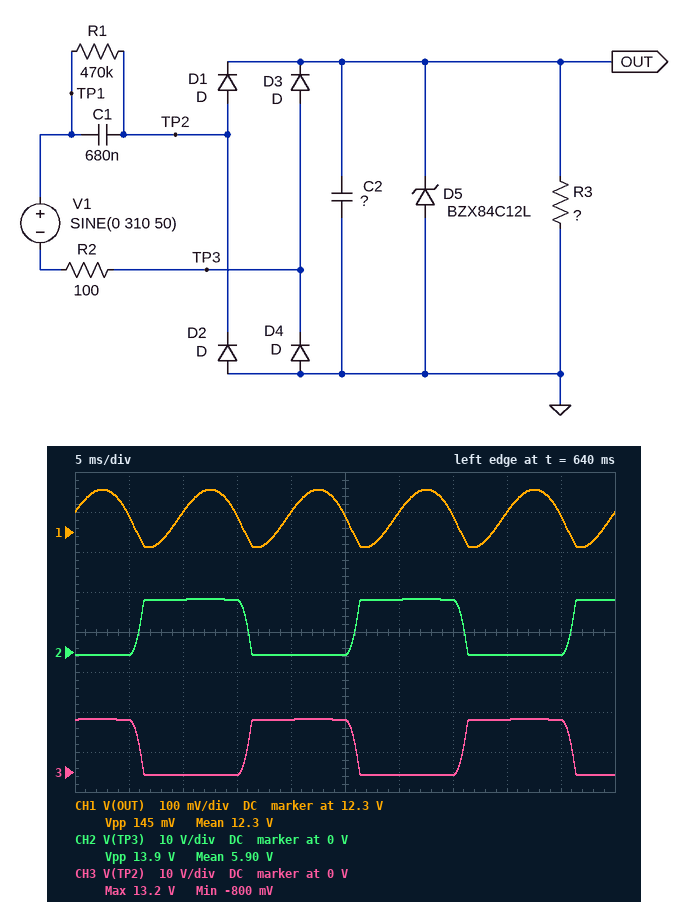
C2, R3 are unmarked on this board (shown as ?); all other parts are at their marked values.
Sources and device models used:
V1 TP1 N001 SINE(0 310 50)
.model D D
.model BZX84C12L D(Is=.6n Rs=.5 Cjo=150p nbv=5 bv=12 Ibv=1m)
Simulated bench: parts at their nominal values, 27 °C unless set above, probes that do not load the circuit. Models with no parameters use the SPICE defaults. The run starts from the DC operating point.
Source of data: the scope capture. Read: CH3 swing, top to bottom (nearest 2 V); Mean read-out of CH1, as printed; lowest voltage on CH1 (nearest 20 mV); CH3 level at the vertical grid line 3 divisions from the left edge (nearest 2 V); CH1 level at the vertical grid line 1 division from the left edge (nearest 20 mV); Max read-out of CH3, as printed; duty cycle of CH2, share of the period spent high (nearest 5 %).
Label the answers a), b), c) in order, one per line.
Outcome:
a) 14 V
b) 12.3 V
c) 12.26 V
d) 0 V
e) 12.34 V
f) 13.2 V
g) 50 %
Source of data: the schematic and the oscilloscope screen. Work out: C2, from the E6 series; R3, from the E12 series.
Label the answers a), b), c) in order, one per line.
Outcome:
a) 680 µF
b) 470 Ω
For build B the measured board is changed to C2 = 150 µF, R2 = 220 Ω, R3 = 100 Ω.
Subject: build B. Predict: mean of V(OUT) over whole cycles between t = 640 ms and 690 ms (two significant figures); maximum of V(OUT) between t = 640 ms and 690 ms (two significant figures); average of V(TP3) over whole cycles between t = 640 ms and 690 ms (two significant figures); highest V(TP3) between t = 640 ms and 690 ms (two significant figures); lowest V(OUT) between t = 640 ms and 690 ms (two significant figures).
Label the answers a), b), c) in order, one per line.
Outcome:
a) 4.1 V
b) 4.4 V
c) 2.1 V
d) 5.2 V
e) 3.8 V
